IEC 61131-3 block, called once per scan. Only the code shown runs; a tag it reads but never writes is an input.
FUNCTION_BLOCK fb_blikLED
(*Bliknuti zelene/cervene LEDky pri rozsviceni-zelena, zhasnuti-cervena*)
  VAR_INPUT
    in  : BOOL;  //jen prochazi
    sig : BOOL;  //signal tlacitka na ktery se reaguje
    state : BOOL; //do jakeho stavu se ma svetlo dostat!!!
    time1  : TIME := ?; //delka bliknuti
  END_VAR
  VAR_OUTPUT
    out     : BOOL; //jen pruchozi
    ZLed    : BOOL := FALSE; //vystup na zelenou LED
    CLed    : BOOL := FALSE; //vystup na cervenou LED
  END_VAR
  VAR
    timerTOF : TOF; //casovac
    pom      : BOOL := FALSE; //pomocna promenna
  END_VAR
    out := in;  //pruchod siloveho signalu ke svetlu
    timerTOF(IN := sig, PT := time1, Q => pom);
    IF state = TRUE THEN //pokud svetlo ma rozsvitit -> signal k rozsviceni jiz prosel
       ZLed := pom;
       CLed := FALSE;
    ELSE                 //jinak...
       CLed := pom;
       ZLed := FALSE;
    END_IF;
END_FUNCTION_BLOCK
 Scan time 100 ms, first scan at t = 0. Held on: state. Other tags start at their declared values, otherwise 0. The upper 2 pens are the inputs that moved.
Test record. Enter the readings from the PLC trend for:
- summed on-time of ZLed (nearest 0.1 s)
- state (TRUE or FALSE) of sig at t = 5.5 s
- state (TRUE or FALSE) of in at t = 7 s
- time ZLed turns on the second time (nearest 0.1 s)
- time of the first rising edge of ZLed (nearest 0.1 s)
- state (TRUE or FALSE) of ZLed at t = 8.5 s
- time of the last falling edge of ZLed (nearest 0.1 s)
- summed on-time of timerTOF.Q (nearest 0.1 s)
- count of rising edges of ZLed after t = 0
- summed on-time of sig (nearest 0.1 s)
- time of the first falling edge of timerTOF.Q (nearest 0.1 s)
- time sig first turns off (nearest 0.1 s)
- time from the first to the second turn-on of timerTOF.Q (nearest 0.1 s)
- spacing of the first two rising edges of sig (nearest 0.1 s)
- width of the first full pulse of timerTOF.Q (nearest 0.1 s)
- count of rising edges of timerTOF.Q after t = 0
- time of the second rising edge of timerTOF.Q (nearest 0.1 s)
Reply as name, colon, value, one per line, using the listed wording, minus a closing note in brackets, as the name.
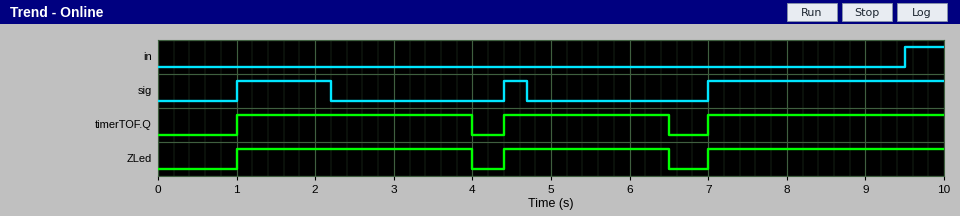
summed on-time of ZLed: 8.1 s
state (TRUE or FALSE) of sig at t = 5.5 s: FALSE
state (TRUE or FALSE) of in at t = 7 s: FALSE
time ZLed turns on the second time: 4.4 s
time of the first rising edge of ZLed: 1.0 s
state (TRUE or FALSE) of ZLed at t = 8.5 s: TRUE
time of the last falling edge of ZLed: 6.5 s
summed on-time of timerTOF.Q: 8.1 s
count of rising edges of ZLed after t = 0: 3
summed on-time of sig: 4.5 s
time of the first falling edge of timerTOF.Q: 4.0 s
time sig first turns off: 2.2 s
time from the first to the second turn-on of timerTOF.Q: 3.4 s
spacing of the first two rising edges of sig: 3.4 s
width of the first full pulse of timerTOF.Q: 3.0 s
count of rising edges of timerTOF.Q after t = 0: 3
time of the second rising edge of timerTOF.Q: 4.4 s
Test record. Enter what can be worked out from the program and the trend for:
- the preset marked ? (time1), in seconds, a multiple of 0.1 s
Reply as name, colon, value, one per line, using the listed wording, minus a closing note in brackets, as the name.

the preset marked ? (time1), in seconds, a multiple of 0.1 s: 1.8 s
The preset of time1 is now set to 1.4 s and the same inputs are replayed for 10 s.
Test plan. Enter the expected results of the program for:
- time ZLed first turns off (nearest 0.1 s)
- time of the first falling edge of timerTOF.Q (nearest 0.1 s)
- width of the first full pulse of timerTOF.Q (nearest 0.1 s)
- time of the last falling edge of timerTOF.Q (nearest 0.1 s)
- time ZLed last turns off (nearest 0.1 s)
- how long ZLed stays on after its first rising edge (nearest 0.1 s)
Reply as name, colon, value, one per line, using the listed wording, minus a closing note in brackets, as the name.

time ZLed first turns off: 3.6 s
time of the first falling edge of timerTOF.Q: 3.6 s
width of the first full pulse of timerTOF.Q: 2.6 s
time of the last falling edge of timerTOF.Q: 6.1 s
time ZLed last turns off: 6.1 s
how long ZLed stays on after its first rising edge: 2.6 s
